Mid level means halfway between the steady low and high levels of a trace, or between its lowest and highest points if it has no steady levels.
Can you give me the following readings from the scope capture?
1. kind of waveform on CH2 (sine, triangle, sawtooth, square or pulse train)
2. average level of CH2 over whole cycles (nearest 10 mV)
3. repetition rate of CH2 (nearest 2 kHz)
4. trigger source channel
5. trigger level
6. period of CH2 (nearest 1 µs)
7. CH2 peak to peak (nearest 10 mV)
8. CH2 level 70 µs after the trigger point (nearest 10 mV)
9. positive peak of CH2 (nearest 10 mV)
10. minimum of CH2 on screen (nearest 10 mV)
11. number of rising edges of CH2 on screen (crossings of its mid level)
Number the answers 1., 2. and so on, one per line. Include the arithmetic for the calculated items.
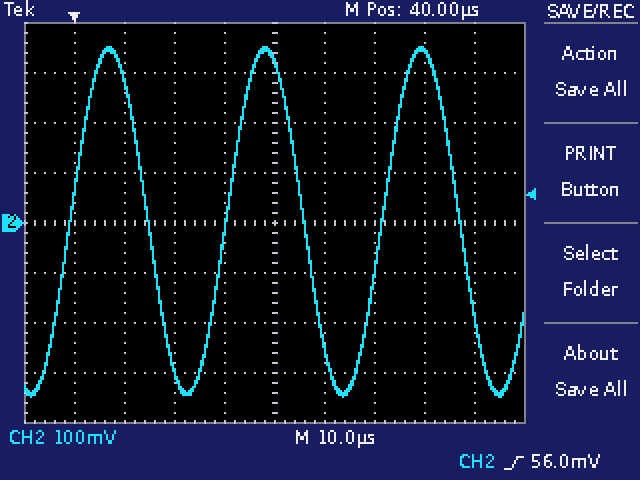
1. sine
2. (350 mV + (-350 mV)) / 2 ≈ 0 mV
3. 1 / 31 µs ≈ 32 kHz
4. CH2
5. 56.0 mV
6. 31 µs
7. 350 mV − (-350 mV) = 700 mV
8. 340 mV
9. 350 mV
10. -350 mV
11. 3
